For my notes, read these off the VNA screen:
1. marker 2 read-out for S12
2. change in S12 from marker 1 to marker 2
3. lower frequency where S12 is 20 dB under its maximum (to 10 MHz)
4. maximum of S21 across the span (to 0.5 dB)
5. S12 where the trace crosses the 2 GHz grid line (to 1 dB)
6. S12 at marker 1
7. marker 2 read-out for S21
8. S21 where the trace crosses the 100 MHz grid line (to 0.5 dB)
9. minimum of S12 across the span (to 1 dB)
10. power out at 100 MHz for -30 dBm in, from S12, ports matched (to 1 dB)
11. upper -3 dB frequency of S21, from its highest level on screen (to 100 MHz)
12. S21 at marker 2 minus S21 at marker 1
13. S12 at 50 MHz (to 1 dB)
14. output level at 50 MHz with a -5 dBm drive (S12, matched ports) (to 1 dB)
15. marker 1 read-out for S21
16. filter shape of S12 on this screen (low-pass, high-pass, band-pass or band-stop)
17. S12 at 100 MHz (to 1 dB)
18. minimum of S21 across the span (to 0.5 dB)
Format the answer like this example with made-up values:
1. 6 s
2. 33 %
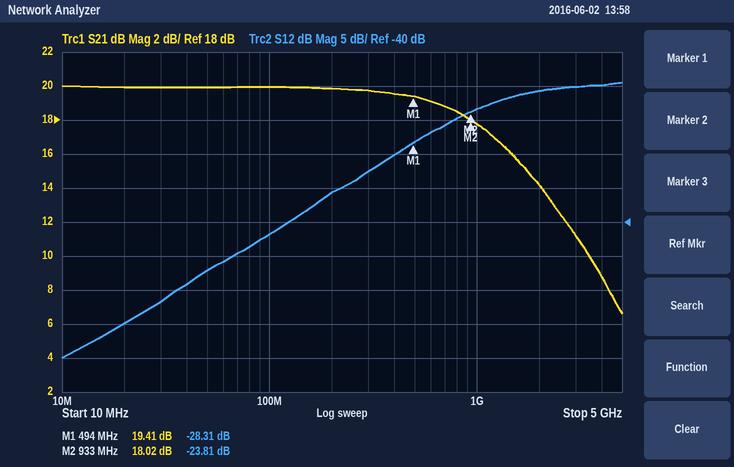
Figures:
1. -23.81 dB
2. 4.50 dB
3. 130 MHz
4. 20.0 dB
5. -21 dB
6. -28.31 dB
7. 18.02 dB
8. 20.0 dB
9. -60 dB
10. -72 dBm
11. 1.2 GHz
12. -1.39 dB
13. -47 dB
14. -52 dBm
15. 19.41 dB
16. high-pass
17. -42 dB
18. 6.5 dB
